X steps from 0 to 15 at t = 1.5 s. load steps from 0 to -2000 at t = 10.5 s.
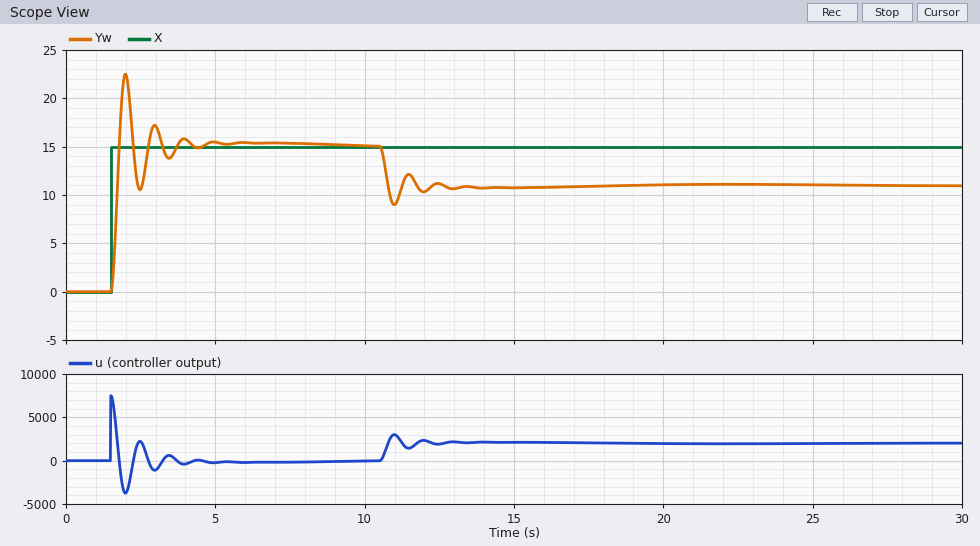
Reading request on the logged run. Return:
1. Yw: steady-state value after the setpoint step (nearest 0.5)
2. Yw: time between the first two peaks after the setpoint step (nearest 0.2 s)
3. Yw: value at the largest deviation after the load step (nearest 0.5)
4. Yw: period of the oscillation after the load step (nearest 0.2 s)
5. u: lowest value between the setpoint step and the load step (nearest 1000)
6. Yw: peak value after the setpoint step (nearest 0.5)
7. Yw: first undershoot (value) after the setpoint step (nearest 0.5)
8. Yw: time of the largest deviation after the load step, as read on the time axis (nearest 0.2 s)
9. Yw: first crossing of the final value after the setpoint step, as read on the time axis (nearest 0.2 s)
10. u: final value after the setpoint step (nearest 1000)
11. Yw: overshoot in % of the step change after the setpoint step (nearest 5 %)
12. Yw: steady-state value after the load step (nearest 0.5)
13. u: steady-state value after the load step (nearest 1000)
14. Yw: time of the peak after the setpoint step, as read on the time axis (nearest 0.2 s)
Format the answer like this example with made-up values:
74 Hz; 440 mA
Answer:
15.0; 1.0 s; 9.0; 1.0 s; -4000; 22.5; 10.5; 11.0 s; 1.8 s; 0; 50 %; 11.0; 2000; 2.0 s
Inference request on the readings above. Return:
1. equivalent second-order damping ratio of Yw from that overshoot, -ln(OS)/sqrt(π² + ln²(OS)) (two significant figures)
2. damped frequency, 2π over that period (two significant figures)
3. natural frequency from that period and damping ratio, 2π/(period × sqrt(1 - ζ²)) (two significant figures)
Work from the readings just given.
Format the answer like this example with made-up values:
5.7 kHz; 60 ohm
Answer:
0.22; 6.3 rad/s; 6.4 rad/s
